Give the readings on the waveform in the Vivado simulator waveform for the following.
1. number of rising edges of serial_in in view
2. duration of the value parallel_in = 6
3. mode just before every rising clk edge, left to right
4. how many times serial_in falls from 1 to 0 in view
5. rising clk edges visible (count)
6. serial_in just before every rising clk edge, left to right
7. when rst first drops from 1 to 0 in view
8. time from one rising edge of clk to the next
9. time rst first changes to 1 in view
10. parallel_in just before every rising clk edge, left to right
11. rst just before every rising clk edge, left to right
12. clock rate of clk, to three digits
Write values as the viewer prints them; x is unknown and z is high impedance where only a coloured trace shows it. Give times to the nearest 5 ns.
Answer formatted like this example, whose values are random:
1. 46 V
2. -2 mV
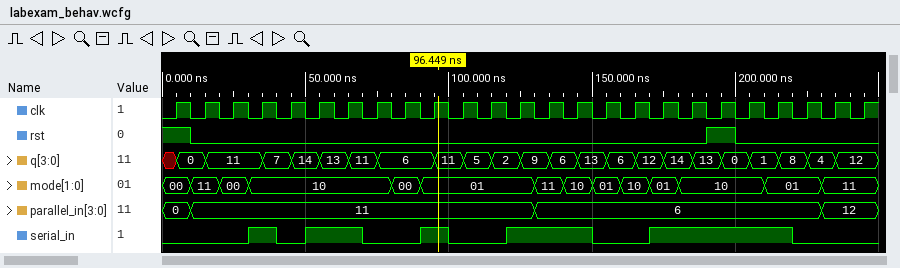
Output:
1. 5
2. 100 ns
3. 00, 11, 00, 10, 10, 10, 10, 10, 00, 01, 01, 01, 01, 11, 10, 01, 10, 01, 10, 10, 10, 01, 01, 11, 11
4. 5
5. 25
6. 0 0 0 1 0 1 1 0 0 1 0 0 1 1 1 0 0 1 1 1 1 1 0 0 0
7. 10 ns
8. 10 ns
9. 190 ns
10. 0, 11, 11, 11, 11, 11, 11, 11, 11, 11, 11, 11, 11, 6, 6, 6, 6, 6, 6, 6, 6, 6, 6, 12, 12
11. 1 0 0 0 0 0 0 0 0 0 0 0 0 0 0 0 0 0 0 1 0 0 0 0 0
12. 100 MHz
